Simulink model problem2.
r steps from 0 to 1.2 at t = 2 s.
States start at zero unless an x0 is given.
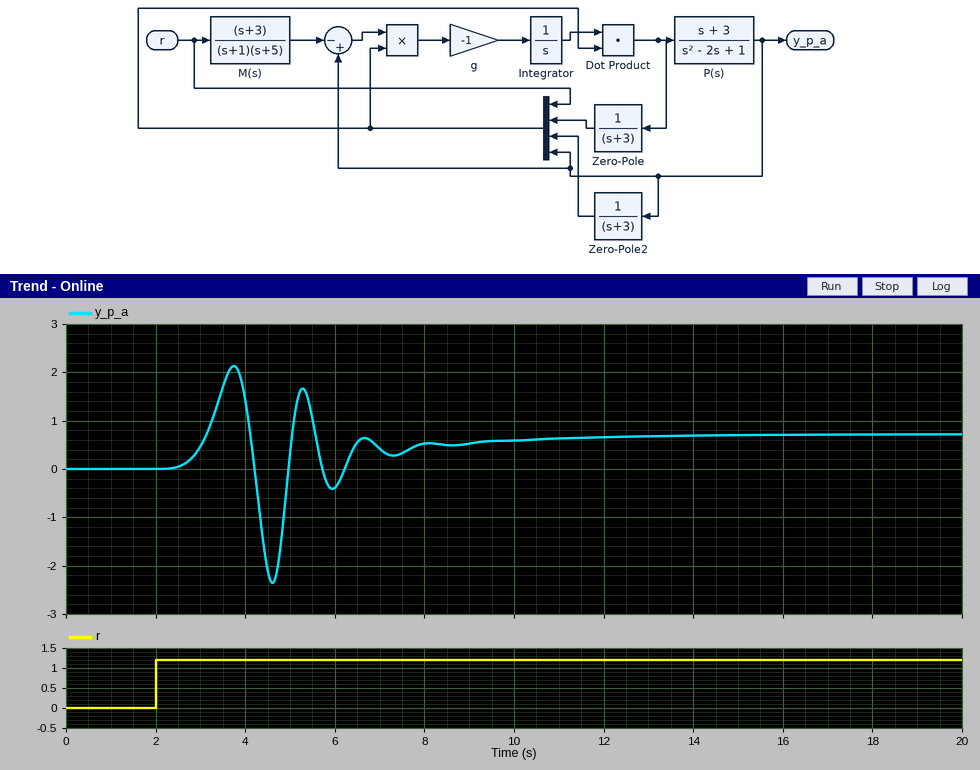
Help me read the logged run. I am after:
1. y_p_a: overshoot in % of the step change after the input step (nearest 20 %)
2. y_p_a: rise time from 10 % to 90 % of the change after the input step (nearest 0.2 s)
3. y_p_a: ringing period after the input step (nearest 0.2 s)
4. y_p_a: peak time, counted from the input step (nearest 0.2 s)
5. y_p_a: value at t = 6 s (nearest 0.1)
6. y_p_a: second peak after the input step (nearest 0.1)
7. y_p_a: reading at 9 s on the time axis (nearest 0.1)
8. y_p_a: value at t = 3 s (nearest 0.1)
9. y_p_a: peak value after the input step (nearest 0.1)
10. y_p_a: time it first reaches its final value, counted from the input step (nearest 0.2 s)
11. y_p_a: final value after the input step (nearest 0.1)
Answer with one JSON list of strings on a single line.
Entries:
["200 %", "0.6 s", "1.6 s", "1.8 s", "-0.4", "1.7", "0.5", "0.5", "2.1", "1.2 s", "0.7"]
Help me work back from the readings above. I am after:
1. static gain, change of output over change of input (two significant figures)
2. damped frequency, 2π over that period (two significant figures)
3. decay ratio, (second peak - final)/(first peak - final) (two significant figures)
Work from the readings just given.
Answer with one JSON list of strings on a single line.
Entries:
["0.58", "3.9 rad/s", "0.71"]
